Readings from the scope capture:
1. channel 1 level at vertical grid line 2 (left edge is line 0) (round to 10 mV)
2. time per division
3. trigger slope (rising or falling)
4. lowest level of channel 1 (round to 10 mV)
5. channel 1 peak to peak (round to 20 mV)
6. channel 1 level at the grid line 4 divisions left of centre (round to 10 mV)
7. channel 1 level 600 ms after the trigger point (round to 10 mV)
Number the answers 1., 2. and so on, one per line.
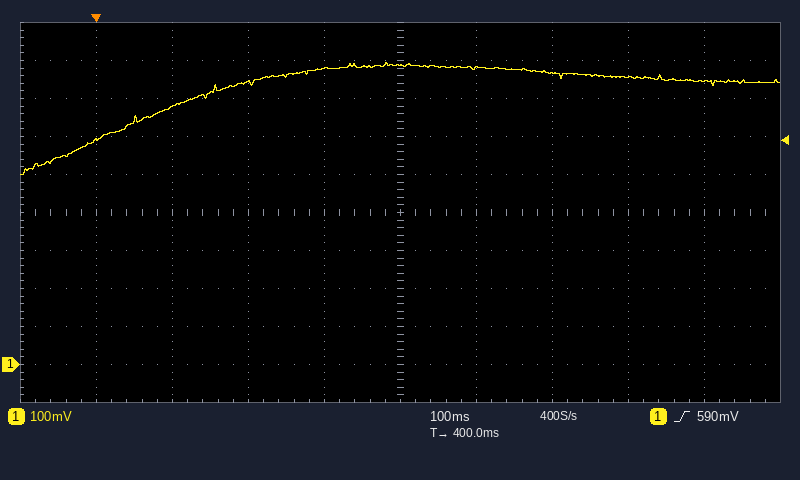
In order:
1. 680 mV
2. 100 ms
3. rising
4. 500 mV
5. 300 mV
6. 590 mV
7. 770 mV
